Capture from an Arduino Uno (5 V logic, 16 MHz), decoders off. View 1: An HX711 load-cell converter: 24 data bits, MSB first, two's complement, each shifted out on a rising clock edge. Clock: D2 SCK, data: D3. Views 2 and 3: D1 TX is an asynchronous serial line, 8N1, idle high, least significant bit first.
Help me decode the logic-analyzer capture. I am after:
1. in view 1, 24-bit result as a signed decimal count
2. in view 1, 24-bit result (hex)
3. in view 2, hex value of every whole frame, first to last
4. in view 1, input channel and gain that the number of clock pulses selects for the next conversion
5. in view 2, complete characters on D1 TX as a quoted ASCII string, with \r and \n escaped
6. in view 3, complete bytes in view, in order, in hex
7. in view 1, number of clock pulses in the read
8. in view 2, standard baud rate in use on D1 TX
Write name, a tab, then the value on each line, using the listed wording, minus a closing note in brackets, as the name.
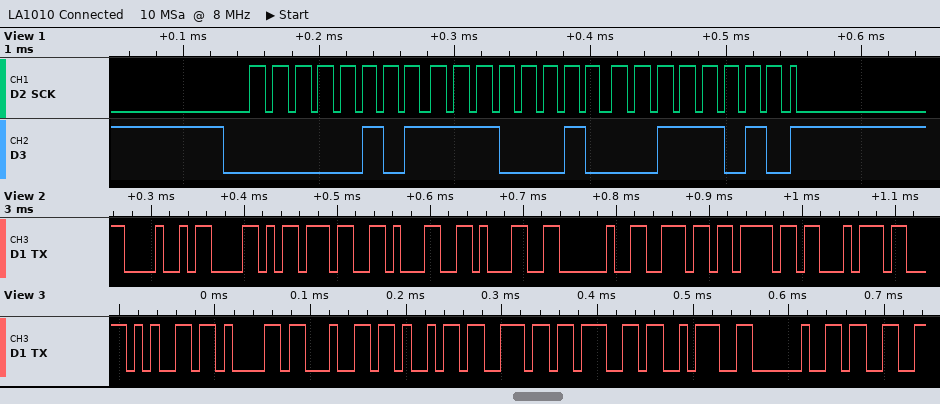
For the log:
in view 1, 24-bit result as a signed decimal count	385594
in view 1, 24-bit result	0x05E23A
in view 2, hex value of every whole frame, first to last	48 58 37 31 31 20 6E 6F 74
in view 1, input channel and gain that the number of clock pulses selects for the next conversion	channel A, gain 128
in view 2, complete characters on D1 TX as a quoted ASCII string, with \r and \n escaped	"HX711 not"
in view 3, complete bytes in view, in order, in hex	65 61 64 69 6E 67 3A 20 33
in view 1, number of clock pulses in the read	25
in view 2, standard baud rate in use on D1 TX	115200 baud
